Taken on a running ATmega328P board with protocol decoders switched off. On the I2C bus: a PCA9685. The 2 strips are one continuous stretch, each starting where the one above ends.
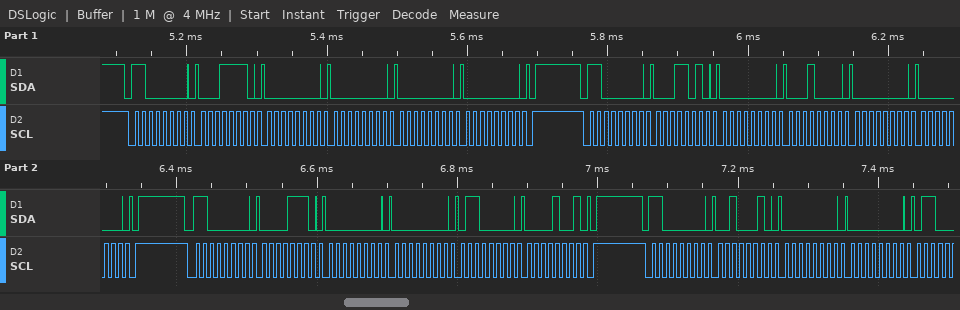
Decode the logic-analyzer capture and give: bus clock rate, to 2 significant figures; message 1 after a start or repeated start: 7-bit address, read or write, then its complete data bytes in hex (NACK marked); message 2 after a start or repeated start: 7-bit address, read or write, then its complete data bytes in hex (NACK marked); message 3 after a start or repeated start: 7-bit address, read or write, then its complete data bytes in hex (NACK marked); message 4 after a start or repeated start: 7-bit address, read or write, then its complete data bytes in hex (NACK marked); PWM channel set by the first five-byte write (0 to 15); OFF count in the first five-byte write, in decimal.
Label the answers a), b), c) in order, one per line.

a) 100 kHz
b) 0x60 write: 1E 00 00 00 00
c) 0x60 write: 1A 00 10 00 00
d) 0x60 write: 0E 00 00 60 09
e) 0x60 write: 22 00 00
f) 6
g) 0
